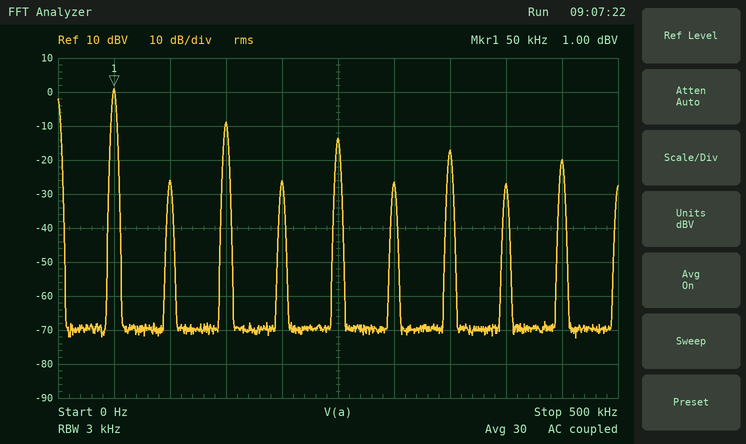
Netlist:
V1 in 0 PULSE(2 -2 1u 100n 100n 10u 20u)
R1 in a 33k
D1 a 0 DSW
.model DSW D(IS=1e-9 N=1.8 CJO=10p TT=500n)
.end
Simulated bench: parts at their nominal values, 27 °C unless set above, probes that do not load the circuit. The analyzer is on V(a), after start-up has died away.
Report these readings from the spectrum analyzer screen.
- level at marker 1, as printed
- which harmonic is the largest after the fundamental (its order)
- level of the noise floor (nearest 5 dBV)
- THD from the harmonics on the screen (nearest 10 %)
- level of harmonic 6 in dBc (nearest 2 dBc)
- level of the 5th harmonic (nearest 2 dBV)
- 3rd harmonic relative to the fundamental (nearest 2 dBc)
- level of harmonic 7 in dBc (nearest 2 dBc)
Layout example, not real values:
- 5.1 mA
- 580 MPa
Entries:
- 1.00 dBV
- 3
- -70 dBV
- 40 %
- -28 dBc
- -14 dBV
- -10 dBc
- -18 dBc
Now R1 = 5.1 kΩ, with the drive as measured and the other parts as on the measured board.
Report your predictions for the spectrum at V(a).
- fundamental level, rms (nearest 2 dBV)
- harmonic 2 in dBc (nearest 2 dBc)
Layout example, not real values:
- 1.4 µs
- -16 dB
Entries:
- 2 dBV
- -34 dBc
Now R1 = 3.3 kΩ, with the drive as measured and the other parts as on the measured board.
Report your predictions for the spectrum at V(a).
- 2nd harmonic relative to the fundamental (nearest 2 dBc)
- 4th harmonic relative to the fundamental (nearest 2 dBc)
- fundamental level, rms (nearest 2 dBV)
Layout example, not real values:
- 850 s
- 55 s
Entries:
- -34 dBc
- -34 dBc
- 2 dBV
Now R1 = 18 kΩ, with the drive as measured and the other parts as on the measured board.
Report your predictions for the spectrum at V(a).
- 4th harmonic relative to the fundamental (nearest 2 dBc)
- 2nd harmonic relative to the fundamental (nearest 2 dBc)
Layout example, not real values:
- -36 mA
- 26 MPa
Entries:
- -30 dBc
- -30 dBc
